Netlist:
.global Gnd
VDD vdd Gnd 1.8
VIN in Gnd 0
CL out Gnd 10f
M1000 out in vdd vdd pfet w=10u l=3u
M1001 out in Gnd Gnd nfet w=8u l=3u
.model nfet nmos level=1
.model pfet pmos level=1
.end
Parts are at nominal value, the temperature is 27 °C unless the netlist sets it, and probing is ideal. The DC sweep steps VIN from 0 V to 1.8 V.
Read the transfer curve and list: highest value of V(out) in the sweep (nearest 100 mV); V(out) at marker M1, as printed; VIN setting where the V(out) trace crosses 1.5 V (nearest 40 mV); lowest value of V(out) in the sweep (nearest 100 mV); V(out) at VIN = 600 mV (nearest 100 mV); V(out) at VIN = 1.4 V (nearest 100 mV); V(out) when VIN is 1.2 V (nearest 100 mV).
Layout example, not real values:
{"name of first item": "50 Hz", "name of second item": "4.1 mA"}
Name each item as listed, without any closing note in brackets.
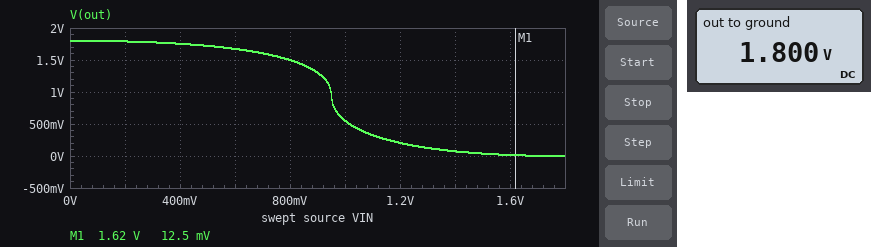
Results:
{"highest value of V(out) in the sweep": "1.8 V", "V(out) at marker M1, as printed": "12.5 mV", "VIN setting where the V(out) trace crosses 1.5 V": "800 mV", "lowest value of V(out) in the sweep": "0 V", "V(out) at VIN = 600 mV": "1.7 V", "V(out) at VIN = 1.4 V": "100 mV", "V(out) when VIN is 1.2 V": "200 mV"}
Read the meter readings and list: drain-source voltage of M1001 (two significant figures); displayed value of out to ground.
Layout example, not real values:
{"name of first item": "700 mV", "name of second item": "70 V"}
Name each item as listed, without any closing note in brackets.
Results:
{"drain-source voltage of M1001": "1.8 V", "displayed value of out to ground": "1.800 V"}
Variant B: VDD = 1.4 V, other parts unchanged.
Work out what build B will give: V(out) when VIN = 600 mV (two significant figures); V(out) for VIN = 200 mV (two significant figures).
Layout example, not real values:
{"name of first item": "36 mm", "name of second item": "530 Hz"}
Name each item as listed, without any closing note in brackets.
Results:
{"V(out) when VIN = 600 mV": "1.2 V", "V(out) for VIN = 200 mV": "1.4 V"}
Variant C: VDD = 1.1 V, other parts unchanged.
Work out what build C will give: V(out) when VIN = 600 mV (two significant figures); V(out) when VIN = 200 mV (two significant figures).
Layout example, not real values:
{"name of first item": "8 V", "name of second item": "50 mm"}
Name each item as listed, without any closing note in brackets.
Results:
{"V(out) when VIN = 600 mV": "380 mV", "V(out) when VIN = 200 mV": "1.1 V"}
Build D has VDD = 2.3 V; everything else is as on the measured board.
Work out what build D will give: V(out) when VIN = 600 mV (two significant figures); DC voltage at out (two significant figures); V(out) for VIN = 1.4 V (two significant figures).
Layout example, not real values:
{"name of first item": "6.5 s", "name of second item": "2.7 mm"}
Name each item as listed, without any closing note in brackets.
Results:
{"V(out) when VIN = 600 mV": "2.2 V", "DC voltage at out": "2.3 V", "V(out) for VIN = 1.4 V": "430 mV"}
